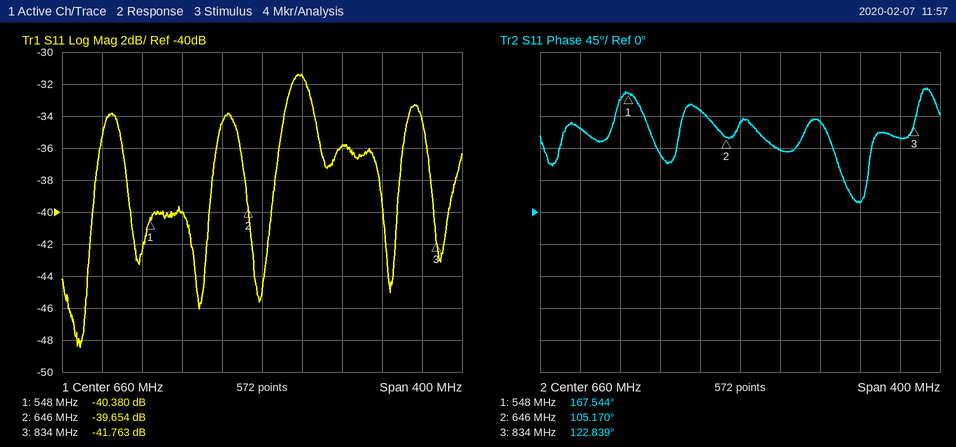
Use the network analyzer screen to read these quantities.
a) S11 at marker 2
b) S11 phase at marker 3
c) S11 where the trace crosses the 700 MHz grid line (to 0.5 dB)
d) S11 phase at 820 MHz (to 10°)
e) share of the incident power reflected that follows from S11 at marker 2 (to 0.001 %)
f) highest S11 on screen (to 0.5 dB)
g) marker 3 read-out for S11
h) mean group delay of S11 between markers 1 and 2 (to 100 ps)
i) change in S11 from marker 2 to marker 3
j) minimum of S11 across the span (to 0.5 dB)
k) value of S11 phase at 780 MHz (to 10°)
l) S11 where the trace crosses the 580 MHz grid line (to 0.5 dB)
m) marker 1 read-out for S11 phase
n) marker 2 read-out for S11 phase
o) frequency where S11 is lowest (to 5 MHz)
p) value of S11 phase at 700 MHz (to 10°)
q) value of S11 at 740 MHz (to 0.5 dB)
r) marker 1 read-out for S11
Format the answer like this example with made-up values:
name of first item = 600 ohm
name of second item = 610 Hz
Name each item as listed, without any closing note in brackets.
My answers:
S11 at marker 2 = -39.654 dB
S11 phase at marker 3 = 122.839°
S11 where the trace crosses the 700 MHz grid line = -31.5 dB
S11 phase at 820 MHz = 100°
share of the incident power reflected that follows from S11 at marker 2 = 0.011 %
highest S11 on screen = -31.5 dB
marker 3 read-out for S11 = -41.763 dB
mean group delay of S11 between markers 1 and 2 = 1.8 ns
change in S11 from marker 2 to marker 3 = -2.109 dB
minimum of S11 across the span = -48.5 dB
value of S11 phase at 780 MHz = 10°
S11 where the trace crosses the 580 MHz grid line = -40.0 dB
marker 1 read-out for S11 phase = 167.544°
marker 2 read-out for S11 phase = 105.170°
frequency where S11 is lowest = 480 MHz
value of S11 phase at 700 MHz = 90°
value of S11 at 740 MHz = -36.0 dB
marker 1 read-out for S11 = -40.380 dB
